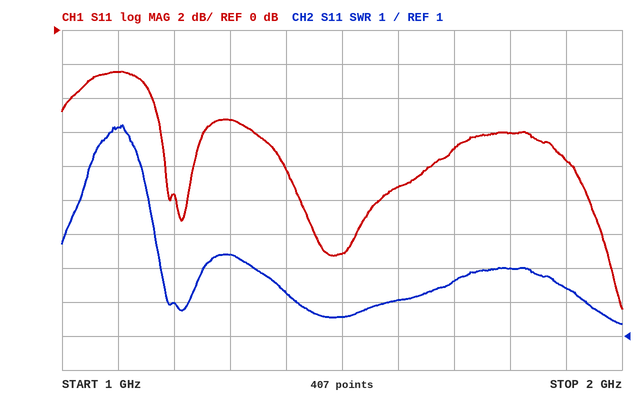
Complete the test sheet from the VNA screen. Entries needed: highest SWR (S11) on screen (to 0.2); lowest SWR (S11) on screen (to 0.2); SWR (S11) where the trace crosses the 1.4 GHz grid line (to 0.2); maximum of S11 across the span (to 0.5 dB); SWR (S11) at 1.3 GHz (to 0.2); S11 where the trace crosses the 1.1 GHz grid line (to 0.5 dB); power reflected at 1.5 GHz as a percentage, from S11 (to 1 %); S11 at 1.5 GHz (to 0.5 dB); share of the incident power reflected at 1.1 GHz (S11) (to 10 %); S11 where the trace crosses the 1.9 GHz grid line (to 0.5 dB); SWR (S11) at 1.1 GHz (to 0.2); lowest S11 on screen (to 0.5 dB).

7.2
1.4
2.2
-2.5 dB
3.4
-2.5 dB
5 %
-13.0 dB
60 %
-7.5 dB
7.2
-16.5 dB
